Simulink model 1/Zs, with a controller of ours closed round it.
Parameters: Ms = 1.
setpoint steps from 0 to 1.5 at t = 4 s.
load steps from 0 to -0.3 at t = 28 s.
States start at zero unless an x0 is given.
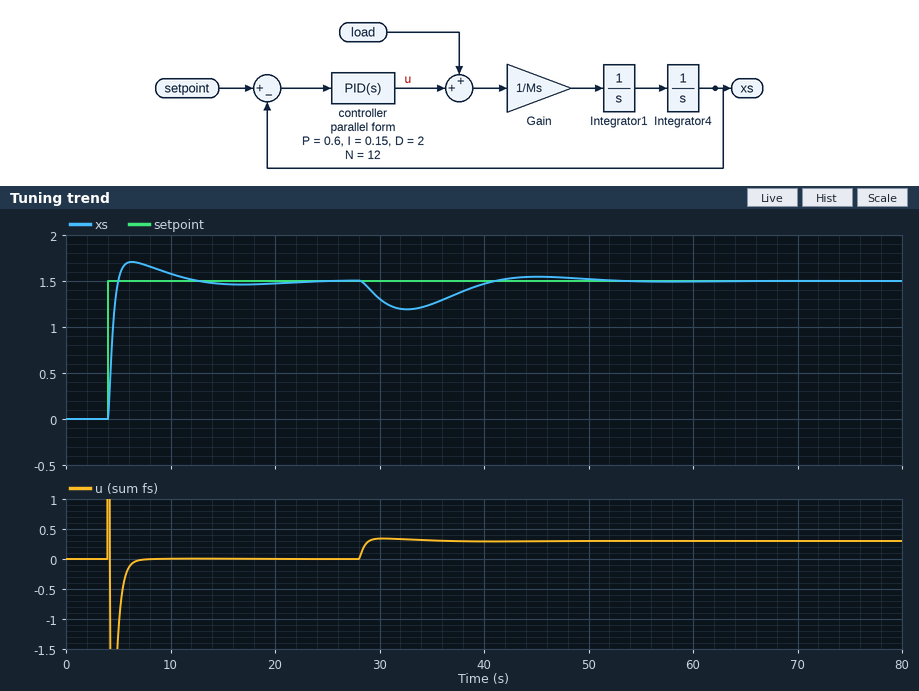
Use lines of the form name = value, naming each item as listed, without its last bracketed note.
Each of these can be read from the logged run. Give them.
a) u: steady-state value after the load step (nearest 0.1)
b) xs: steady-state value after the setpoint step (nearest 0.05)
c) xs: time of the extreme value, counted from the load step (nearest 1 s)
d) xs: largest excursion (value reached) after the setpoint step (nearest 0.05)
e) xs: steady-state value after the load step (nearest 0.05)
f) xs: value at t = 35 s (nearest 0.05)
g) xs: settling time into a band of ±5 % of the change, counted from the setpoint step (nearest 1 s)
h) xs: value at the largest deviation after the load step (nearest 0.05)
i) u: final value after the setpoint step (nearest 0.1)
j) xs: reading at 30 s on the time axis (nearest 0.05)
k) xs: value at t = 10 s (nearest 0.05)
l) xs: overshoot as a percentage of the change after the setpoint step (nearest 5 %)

u: steady-state value after the load step = 0.3
xs: steady-state value after the setpoint step = 1.50
xs: time of the extreme value, counted from the load step = 5 s
xs: largest excursion (value reached) after the setpoint step = 1.70
xs: steady-state value after the load step = 1.50
xs: value at t = 35 s = 1.25
xs: settling time into a band of ±5 % of the change, counted from the setpoint step = 6 s
xs: value at the largest deviation after the load step = 1.20
u: final value after the setpoint step = 0.0
xs: reading at 30 s on the time axis = 1.30
xs: value at t = 10 s = 1.60
xs: overshoot as a percentage of the change after the setpoint step = 15 %
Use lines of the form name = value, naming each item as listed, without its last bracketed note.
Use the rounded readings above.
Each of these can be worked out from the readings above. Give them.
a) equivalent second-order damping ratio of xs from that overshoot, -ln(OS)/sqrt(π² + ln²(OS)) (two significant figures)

equivalent second-order damping ratio of xs from that overshoot, -ln(OS)/sqrt(π² + ln²(OS)) = 0.52
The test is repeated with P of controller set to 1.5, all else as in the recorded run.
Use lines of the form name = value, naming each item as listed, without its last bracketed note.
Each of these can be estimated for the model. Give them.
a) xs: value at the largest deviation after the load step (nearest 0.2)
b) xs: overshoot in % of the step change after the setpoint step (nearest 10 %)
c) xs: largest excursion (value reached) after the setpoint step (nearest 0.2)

xs: value at the largest deviation after the load step = 1.4
xs: overshoot in % of the step change after the setpoint step = 20 %
xs: largest excursion (value reached) after the setpoint step = 1.8
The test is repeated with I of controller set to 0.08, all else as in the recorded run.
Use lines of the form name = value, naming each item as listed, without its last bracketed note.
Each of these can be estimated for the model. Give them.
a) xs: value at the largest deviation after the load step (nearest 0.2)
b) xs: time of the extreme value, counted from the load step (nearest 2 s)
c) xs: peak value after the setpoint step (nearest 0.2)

xs: value at the largest deviation after the load step = 1.2
xs: time of the extreme value, counted from the load step = 6 s
xs: peak value after the setpoint step = 1.6
